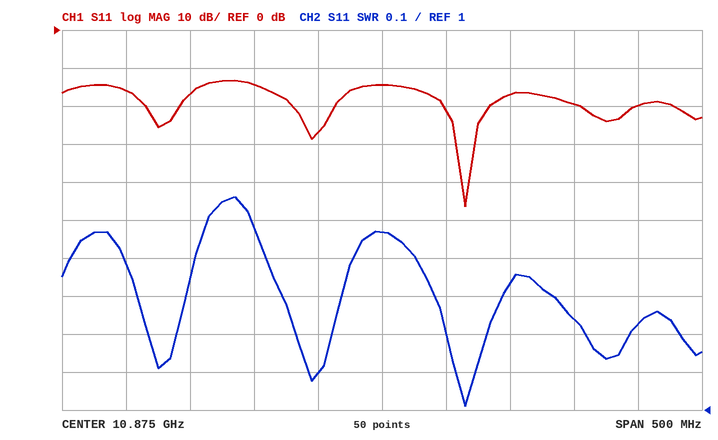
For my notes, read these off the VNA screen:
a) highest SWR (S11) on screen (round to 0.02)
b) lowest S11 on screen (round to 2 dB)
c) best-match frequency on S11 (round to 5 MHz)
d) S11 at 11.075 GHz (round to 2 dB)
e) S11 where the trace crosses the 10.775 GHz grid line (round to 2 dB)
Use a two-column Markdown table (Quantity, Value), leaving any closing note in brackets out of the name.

| Quantity | Value |
|---|---|
| highest SWR (S11) on screen | 1.56 |
| lowest S11 on screen | -46 dB |
| best-match frequency on S11 | 10.940 GHz |
| S11 at 11.075 GHz | -20 dB |
| S11 where the trace crosses the 10.775 GHz grid line | -14 dB |
